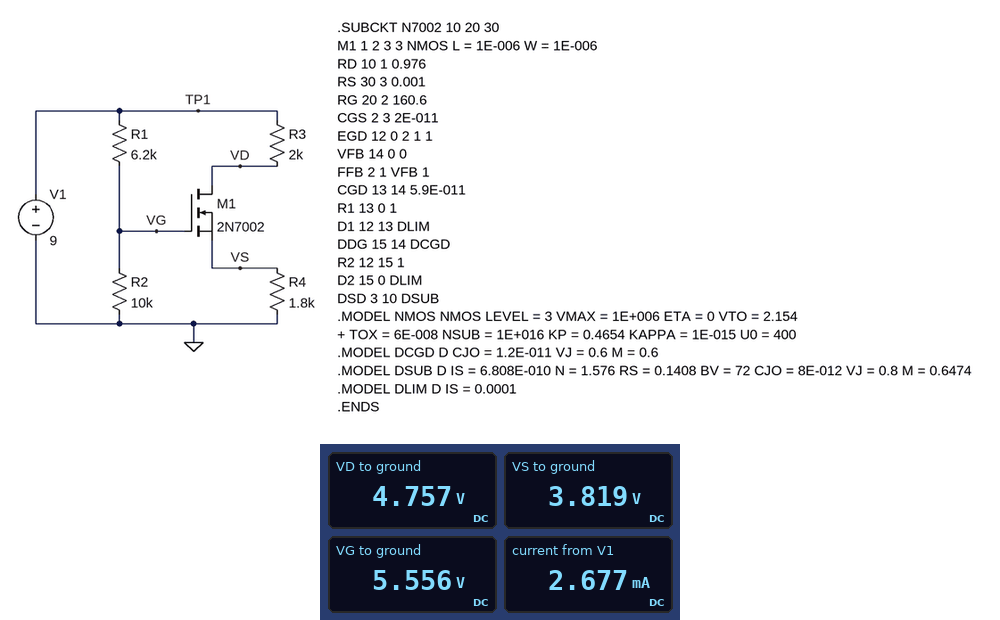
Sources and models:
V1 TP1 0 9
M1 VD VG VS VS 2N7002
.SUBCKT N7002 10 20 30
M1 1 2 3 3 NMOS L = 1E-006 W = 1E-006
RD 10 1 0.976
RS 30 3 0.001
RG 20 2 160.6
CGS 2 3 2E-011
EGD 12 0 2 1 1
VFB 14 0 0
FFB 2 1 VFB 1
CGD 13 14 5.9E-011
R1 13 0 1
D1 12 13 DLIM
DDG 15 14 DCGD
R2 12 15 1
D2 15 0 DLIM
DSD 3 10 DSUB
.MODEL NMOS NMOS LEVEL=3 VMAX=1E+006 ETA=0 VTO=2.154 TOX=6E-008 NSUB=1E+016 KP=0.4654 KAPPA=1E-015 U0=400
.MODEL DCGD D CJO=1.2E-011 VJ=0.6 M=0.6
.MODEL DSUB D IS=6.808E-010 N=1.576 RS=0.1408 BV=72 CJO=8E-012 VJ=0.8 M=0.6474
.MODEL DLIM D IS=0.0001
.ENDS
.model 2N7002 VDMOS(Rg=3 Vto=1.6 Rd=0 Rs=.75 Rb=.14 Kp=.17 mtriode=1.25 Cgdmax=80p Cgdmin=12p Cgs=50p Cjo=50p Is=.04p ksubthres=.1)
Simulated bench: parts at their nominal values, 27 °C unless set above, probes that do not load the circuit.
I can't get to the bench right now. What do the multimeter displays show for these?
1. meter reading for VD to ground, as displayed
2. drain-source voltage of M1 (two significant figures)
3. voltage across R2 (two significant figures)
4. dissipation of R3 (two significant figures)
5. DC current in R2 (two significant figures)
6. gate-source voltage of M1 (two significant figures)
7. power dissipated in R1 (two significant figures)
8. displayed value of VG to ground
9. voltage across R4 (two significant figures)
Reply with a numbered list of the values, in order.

1. 4.757 V
2. 940 mV
3. 5.6 V
4. 9.0 mW
5. 560 µA
6. 1.7 V
7. 1.9 mW
8. 5.556 V
9. 3.8 V
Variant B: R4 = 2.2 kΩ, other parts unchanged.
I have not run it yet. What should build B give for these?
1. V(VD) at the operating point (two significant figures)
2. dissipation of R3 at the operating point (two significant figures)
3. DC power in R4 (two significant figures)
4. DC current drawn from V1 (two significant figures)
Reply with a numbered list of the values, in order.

1. 5.5 V
2. 6.1 mW
3. 6.7 mW
4. 2.3 mA
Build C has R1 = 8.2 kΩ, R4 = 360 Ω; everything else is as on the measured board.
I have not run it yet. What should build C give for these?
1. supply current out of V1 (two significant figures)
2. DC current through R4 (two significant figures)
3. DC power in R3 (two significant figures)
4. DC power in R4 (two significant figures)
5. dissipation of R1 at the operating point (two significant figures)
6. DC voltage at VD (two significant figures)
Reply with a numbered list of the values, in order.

1. 4.3 mA
2. 3.8 mA
3. 29 mW
4. 5.2 mW
5. 2.0 mW
6. 1.4 V
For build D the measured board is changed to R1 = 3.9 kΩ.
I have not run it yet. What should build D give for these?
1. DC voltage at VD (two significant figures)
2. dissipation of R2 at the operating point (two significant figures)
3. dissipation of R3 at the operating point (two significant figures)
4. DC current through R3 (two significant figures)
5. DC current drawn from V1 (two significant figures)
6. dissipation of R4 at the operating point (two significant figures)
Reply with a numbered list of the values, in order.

1. 4.3 V
2. 4.2 mW
3. 11 mW
4. 2.4 mA
5. 3.0 mA
6. 10 mW
